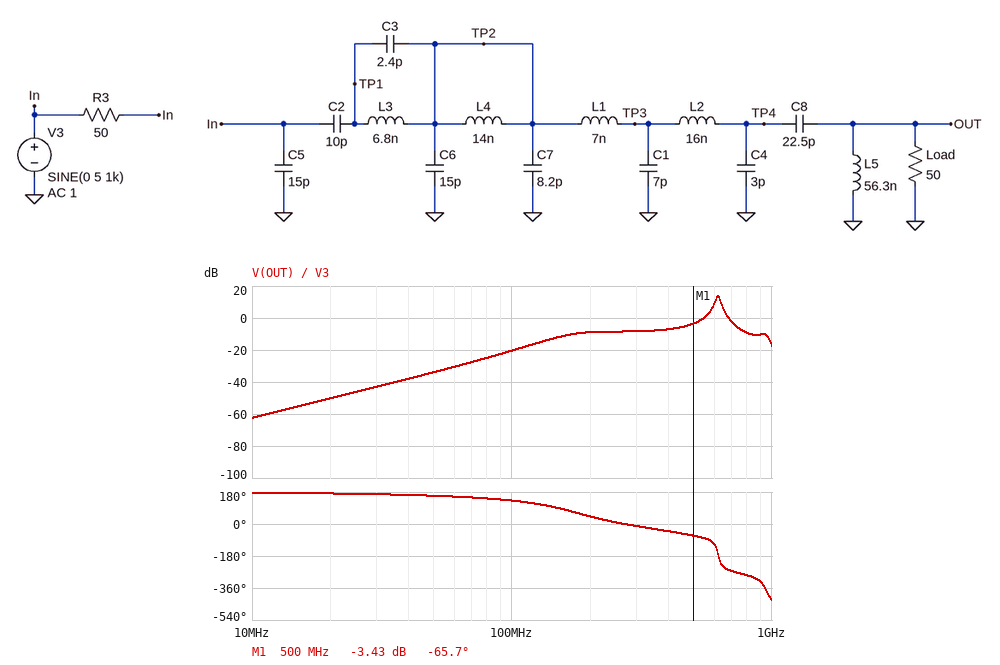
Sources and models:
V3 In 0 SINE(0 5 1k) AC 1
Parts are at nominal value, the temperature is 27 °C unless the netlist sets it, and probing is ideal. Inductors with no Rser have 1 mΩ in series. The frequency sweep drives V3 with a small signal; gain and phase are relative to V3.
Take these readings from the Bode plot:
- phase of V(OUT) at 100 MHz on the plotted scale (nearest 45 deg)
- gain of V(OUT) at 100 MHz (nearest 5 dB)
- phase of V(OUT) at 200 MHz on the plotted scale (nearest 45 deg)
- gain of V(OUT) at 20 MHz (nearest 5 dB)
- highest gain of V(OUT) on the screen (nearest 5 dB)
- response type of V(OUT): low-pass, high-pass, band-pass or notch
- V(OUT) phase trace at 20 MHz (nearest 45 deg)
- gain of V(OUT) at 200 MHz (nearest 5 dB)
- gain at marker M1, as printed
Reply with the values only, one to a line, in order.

135 deg
-20 dB
45 deg
-50 dB
15 dB
band-pass
180 deg
-10 dB
-3.43 dB
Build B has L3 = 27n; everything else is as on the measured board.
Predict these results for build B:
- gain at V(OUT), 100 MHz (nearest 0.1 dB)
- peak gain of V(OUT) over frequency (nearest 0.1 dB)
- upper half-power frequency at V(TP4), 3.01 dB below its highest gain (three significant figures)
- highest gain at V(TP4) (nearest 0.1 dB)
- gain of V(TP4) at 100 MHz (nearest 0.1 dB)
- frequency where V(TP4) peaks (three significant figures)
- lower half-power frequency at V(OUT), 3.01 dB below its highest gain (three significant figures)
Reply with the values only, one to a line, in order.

-19.7 dB
7.2 dB
327 MHz
6.4 dB
-14.9 dB
312 MHz
294 MHz
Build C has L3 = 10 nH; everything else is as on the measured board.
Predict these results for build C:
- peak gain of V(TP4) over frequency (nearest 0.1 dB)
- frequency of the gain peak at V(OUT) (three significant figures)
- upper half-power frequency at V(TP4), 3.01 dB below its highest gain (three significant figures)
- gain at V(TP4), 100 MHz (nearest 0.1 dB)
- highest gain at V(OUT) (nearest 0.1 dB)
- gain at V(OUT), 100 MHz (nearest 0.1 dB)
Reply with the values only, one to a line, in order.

11.8 dB
514 MHz
527 MHz
-15.5 dB
12.1 dB
-20.3 dB
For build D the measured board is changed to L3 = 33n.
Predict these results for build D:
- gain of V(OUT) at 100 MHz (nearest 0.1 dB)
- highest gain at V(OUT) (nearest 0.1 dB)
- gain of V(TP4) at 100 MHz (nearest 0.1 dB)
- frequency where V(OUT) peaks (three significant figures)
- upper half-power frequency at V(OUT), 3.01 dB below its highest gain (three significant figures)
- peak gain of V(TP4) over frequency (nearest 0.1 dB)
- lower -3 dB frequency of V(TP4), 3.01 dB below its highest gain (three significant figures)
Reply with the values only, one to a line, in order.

-19.5 dB
6.1 dB
-14.7 dB
281 MHz
297 MHz
5.2 dB
262 MHz
